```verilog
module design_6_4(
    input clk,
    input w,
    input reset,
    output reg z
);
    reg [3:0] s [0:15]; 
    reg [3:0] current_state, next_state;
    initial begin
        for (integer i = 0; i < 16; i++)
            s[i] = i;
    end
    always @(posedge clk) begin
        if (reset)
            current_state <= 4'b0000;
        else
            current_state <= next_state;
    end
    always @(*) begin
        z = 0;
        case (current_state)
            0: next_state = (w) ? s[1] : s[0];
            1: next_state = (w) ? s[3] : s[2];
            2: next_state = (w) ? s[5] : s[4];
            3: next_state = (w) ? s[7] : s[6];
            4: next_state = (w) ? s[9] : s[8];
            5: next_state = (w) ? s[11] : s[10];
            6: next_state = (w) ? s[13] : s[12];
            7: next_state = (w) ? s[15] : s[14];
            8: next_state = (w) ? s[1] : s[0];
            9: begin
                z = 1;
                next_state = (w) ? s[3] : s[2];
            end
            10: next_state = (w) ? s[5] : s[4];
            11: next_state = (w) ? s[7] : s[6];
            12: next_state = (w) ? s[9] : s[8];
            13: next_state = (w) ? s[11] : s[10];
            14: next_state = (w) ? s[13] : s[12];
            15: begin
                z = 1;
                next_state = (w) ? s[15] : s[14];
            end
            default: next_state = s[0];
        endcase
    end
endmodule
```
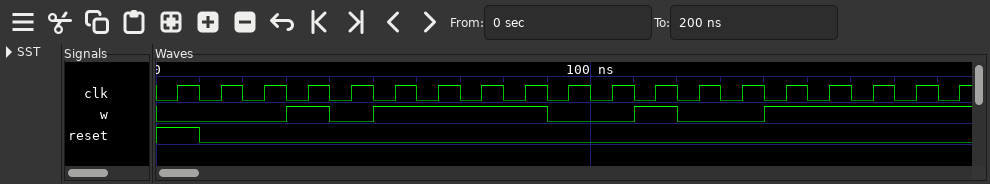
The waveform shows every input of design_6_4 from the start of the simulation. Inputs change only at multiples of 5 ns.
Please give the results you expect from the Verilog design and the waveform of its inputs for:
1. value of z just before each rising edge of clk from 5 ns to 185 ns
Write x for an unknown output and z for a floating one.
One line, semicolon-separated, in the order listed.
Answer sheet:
0 0 0 0 0 0 0 0 0 1 0 0 1 0 0 1 0 0 1
